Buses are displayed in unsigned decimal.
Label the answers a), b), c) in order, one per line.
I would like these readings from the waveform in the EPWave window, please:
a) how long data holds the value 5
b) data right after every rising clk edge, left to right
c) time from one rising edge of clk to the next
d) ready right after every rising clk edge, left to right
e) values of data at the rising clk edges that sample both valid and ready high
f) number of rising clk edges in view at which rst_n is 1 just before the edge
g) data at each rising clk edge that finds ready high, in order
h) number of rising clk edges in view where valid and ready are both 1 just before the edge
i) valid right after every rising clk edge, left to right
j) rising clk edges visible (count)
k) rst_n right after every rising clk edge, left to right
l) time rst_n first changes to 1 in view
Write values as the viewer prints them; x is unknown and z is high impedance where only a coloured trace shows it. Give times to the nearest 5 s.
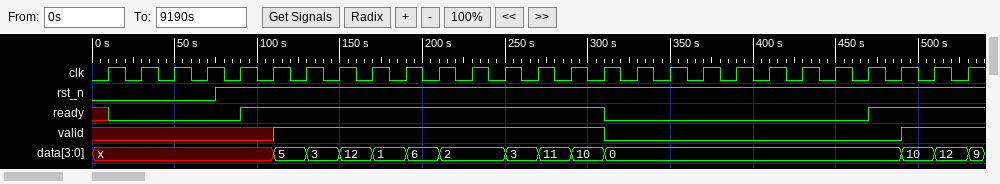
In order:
a) 20 s
b) x, x, x, x, x, 5, 3, 12, 1, 6, 2, 2, 3, 11, 10, 0, 0, 0, 0, 0, 0, 0, 0, 0, 10, 12, 9
c) 20 s
d) 0 0 0 0 1 1 1 1 1 1 1 1 1 1 1 0 0 0 0 0 0 0 0 1 1 1 1
e) 5, 3, 12, 1, 6, 2, 2, 3, 11, 10, 10, 12
f) 23
g) x, 5, 3, 12, 1, 6, 2, 2, 3, 11, 10, 0, 10, 12
h) 12
i) x x x x x 1 1 1 1 1 1 1 1 1 1 0 0 0 0 0 0 0 0 0 1 1 1
j) 27
k) 0 0 0 0 1 1 1 1 1 1 1 1 1 1 1 1 1 1 1 1 1 1 1 1 1 1 1
l) 75 s
